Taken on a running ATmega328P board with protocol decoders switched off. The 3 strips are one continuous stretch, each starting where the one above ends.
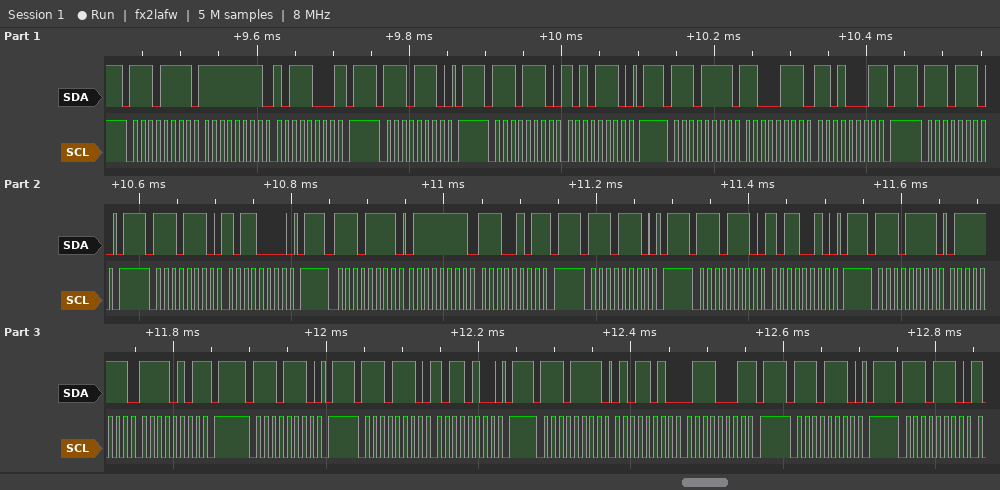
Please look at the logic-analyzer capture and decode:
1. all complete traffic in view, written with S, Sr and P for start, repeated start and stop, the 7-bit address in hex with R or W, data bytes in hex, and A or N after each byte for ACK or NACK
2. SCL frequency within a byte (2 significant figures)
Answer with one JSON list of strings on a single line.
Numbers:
["S 77R A FF A B8 N P S 77W A P S 77W A AE A P S 77R A C7 A D1 N P S 77W A P S 77W A B0 A P S 77R A 7F A E5 N P S 77W A P S 77W A B2 A P S 77R A 7F A F5 N P S 77W A P S 77W A B4 A P S 77R A 5A A 71 N P S 77W A P S 77W A", "100 kHz"]
